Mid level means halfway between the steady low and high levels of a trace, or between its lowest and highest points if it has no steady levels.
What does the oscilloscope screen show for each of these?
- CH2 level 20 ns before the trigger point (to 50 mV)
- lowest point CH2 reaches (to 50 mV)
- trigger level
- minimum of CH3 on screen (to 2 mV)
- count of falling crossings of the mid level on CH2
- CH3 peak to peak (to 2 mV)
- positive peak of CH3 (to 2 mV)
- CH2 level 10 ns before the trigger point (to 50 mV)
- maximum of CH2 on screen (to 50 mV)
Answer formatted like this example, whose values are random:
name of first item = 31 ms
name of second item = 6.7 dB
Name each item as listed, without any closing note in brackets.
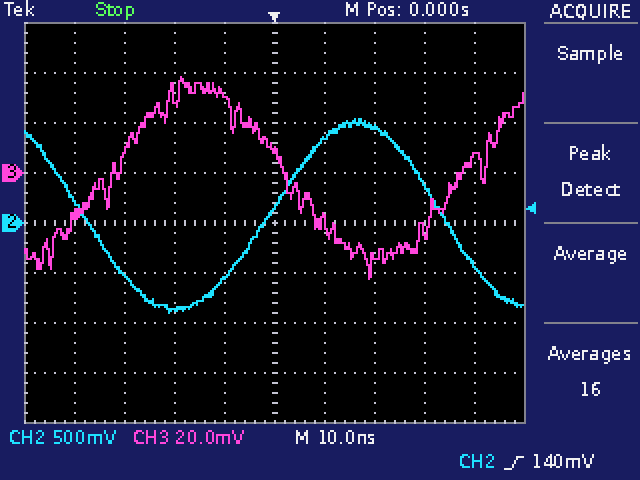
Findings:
CH2 level 20 ns before the trigger point = -850 mV
lowest point CH2 reaches = -900 mV
trigger level = 140 mV
minimum of CH3 on screen = -42 mV
count of falling crossings of the mid level on CH2 = 2
CH3 peak to peak = 80 mV
positive peak of CH3 = 38 mV
CH2 level 10 ns before the trigger point = -550 mV
maximum of CH2 on screen = 1.05 V
